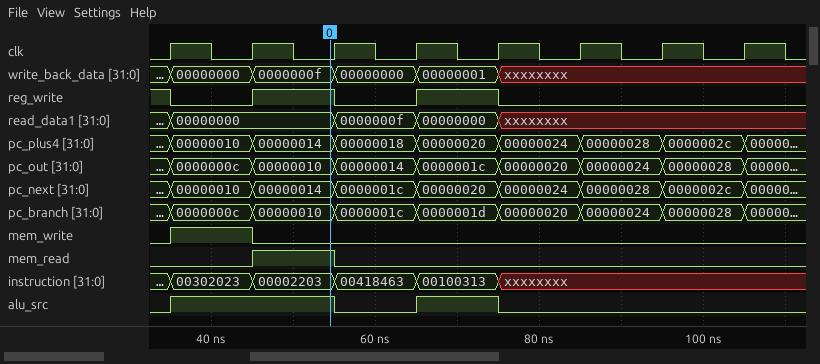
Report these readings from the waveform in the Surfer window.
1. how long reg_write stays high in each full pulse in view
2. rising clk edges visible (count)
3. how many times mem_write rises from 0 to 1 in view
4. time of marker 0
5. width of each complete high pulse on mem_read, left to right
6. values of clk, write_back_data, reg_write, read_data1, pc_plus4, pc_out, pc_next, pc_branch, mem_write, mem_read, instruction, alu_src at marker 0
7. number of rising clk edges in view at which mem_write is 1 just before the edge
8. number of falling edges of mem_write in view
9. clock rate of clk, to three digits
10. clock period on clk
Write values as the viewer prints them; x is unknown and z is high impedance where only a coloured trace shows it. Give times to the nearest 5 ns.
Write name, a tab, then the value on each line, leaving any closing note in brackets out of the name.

how long reg_write stays high in each full pulse in view	10 ns, 10 ns
rising clk edges visible	8
how many times mem_write rises from 0 to 1 in view	1
time of marker 0	55 ns
width of each complete high pulse on mem_read, left to right	10 ns
values of clk, write_back_data, reg_write, read_data1, pc_plus4, pc_out, pc_next, pc_branch, mem_write, mem_read, instruction, alu_src at marker 0	clk=0, write_back_data=0000000f, reg_write=1, read_data1=00000000, pc_plus4=00000014, pc_out=00000010, pc_next=00000014, pc_branch=00000010, mem_write=0, mem_read=1, instruction=00002203, alu_src=1
number of rising clk edges in view at which mem_write is 1 just before the edge	1
number of falling edges of mem_write in view	1
clock rate of clk, to three digits	100 MHz
clock period on clk	10 ns
